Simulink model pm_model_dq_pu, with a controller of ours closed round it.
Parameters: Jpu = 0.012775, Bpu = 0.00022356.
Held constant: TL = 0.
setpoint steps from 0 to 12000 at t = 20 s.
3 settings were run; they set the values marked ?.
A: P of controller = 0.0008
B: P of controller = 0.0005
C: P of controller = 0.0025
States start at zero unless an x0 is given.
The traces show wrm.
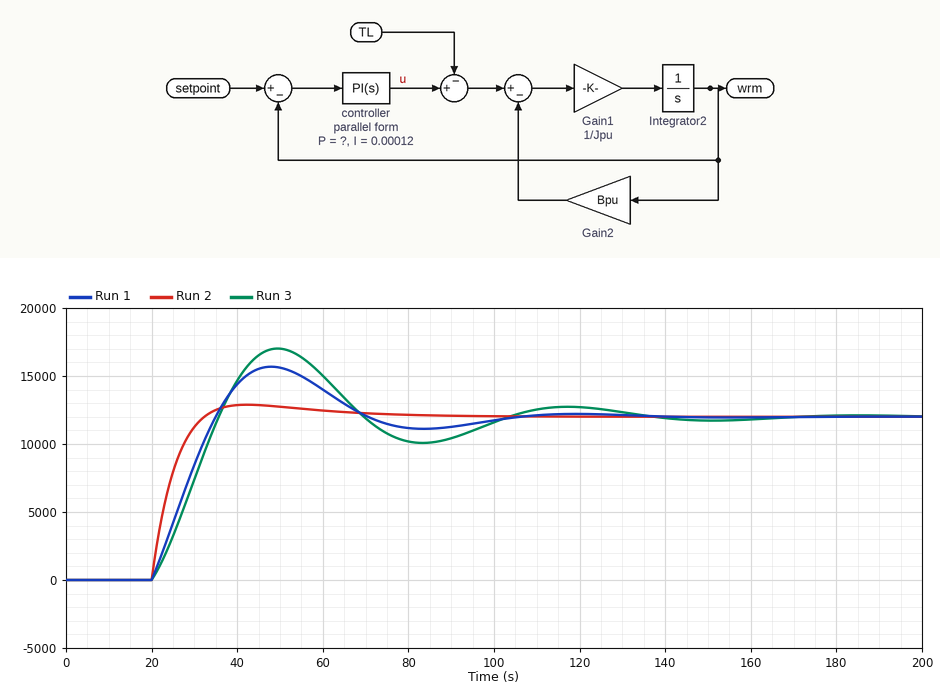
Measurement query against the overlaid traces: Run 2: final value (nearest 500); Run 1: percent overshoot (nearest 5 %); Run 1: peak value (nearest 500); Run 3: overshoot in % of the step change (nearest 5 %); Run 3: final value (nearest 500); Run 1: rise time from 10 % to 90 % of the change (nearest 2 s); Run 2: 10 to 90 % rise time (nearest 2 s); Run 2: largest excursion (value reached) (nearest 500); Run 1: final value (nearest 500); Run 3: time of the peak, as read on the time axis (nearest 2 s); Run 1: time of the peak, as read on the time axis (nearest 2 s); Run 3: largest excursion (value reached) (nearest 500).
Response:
12000
30 %
15500
40 %
12000
12 s
8 s
13000
12000
50 s
48 s
17000
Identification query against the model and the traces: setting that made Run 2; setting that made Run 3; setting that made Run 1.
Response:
C
B
A
